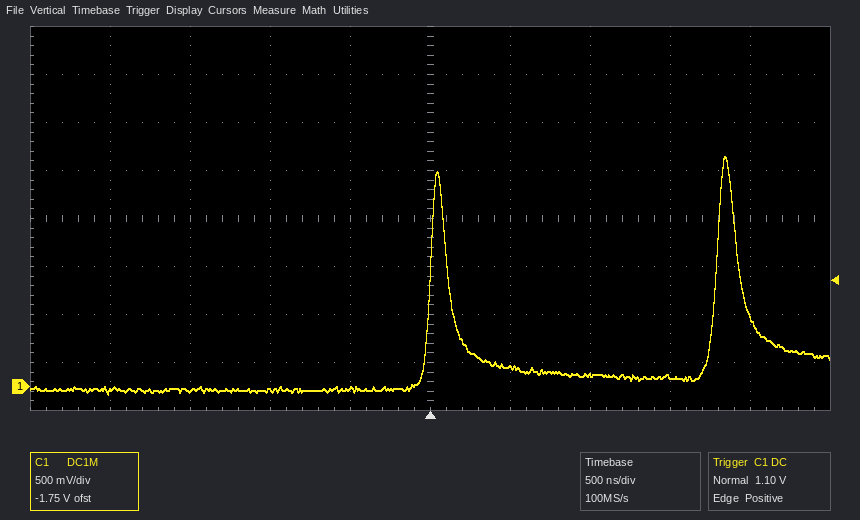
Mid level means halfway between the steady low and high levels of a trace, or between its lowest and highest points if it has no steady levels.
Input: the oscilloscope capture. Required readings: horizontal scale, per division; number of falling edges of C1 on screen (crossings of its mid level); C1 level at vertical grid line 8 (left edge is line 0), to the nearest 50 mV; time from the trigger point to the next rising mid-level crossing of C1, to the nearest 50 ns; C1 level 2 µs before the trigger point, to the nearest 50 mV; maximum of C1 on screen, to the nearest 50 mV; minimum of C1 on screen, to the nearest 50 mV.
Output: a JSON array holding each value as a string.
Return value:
["500 ns", "2", "100 mV", "1.80 µs", "-50 mV", "2.40 V", "-100 mV"]
